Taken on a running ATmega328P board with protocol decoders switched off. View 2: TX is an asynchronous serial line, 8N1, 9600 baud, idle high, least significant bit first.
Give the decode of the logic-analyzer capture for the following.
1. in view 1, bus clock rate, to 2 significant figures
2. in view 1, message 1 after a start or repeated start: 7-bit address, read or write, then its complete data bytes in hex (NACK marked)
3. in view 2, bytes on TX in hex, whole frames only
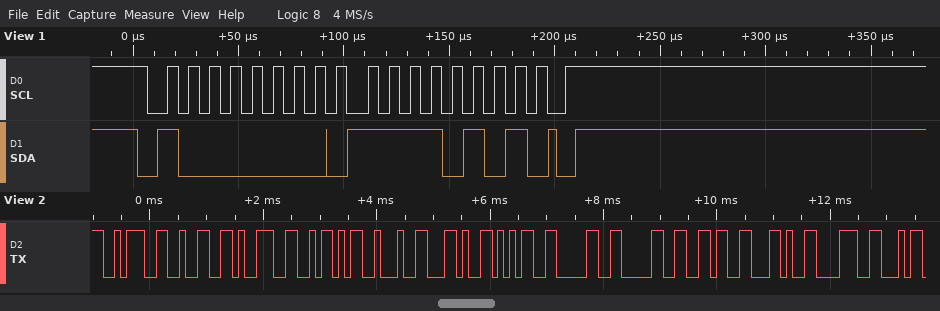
100 kHz
0x40 write: F5
0x3A 0x32 0x39 0x5A 0x22 0x2C 0x35 0x30 0x30 0x36 0x2C 0x38
